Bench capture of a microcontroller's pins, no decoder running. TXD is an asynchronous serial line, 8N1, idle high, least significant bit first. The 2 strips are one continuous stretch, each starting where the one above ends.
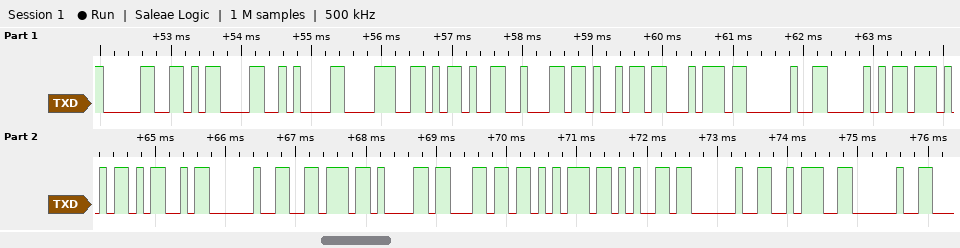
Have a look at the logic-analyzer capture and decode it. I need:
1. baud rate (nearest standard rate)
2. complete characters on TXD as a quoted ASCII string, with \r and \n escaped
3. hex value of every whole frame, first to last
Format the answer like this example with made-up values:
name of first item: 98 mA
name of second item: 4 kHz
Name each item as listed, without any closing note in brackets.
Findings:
baud rate: 9600 baud
complete characters on TXD as a quoted ASCII string, with \r and \n escaped: "0\r\n8-bit PWM value : "
hex value of every whole frame, first to last: 30 0D 0A 38 2D 62 69 74 20 50 57 4D 20 76 61 6C 75 65 20 3A 20
